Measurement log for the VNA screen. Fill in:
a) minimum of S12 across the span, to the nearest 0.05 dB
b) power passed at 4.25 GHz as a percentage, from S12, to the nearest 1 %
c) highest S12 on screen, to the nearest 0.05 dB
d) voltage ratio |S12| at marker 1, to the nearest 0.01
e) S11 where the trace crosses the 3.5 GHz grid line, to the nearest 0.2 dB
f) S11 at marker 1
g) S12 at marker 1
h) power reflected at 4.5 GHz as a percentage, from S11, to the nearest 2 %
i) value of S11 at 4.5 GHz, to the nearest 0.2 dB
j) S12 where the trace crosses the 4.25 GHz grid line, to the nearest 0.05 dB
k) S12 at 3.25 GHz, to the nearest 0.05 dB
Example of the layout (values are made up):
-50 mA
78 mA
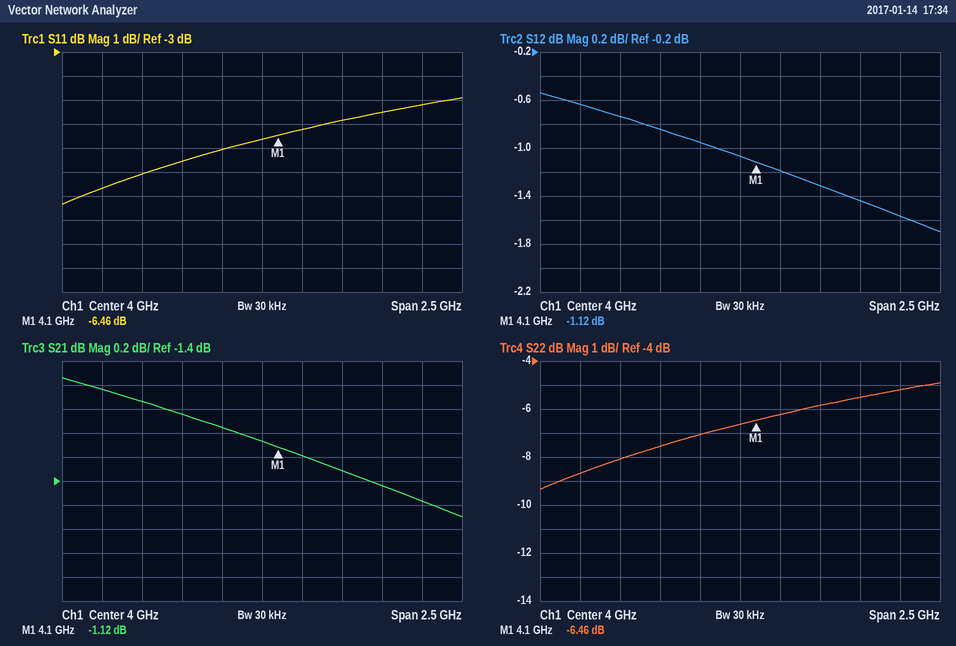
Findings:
-1.70 dB
76 %
-0.55 dB
0.88
-7.6 dB
-6.46 dB
-1.12 dB
26 %
-5.8 dB
-1.20 dB
-0.75 dB
